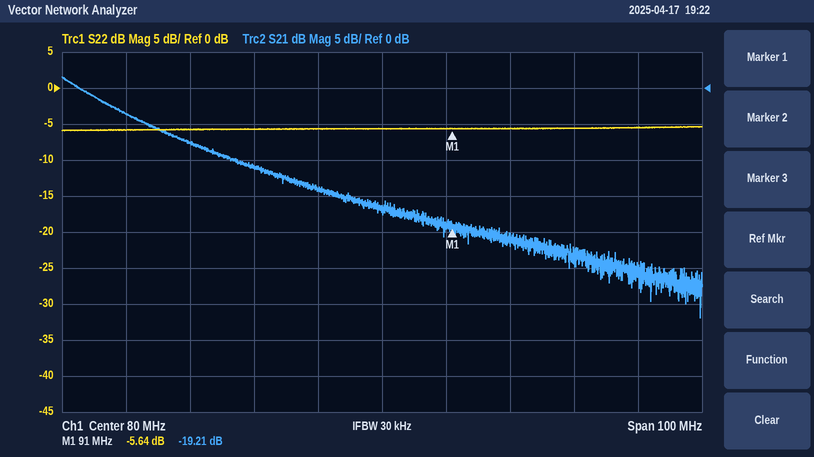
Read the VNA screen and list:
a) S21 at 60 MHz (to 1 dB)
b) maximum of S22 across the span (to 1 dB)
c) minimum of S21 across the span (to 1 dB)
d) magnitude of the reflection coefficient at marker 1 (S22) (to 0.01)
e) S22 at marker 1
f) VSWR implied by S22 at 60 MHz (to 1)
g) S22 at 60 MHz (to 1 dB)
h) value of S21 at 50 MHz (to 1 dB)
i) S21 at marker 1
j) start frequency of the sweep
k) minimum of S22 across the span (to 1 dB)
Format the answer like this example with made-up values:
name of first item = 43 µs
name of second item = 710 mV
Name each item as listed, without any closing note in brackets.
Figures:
S21 at 60 MHz = -11 dB
maximum of S22 across the span = -5 dB
minimum of S21 across the span = -32 dB
magnitude of the reflection coefficient at marker 1 (S22) = 0.52
S22 at marker 1 = -5.64 dB
VSWR implied by S22 at 60 MHz = 3
S22 at 60 MHz = -6 dB
value of S21 at 50 MHz = -8 dB
S21 at marker 1 = -19.21 dB
start frequency of the sweep = 30 MHz
minimum of S22 across the span = -6 dB
